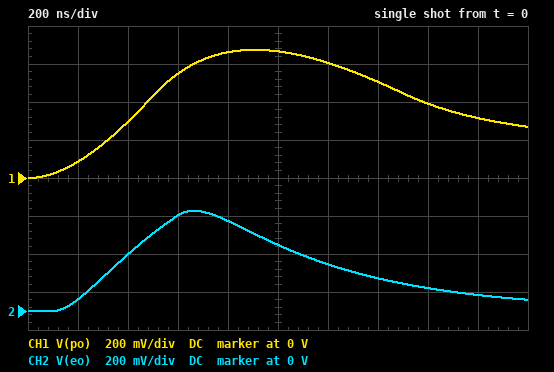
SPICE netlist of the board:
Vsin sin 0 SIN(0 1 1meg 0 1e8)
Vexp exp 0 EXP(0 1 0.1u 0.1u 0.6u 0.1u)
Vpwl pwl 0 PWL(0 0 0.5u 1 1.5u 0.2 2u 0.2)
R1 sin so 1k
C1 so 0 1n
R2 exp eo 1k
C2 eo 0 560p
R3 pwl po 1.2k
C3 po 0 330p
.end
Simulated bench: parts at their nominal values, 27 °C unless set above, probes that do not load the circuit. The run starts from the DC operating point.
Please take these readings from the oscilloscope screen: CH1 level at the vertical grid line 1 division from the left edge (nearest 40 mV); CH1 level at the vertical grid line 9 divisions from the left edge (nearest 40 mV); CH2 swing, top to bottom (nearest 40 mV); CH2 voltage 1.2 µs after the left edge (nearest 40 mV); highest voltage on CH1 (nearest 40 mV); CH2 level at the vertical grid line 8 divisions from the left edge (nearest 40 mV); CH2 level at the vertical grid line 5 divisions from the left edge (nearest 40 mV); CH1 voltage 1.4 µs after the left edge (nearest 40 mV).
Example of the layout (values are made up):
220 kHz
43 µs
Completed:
80 mV
320 mV
520 mV
240 mV
680 mV
120 mV
360 mV
520 mV
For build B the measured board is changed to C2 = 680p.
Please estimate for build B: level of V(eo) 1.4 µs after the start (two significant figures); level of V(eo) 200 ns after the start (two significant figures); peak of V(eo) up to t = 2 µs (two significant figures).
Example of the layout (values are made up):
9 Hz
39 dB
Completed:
190 mV
51 mV
470 mV
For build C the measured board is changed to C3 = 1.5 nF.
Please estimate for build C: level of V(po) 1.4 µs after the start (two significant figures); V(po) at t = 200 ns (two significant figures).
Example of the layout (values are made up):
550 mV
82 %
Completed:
320 mV
21 mV
